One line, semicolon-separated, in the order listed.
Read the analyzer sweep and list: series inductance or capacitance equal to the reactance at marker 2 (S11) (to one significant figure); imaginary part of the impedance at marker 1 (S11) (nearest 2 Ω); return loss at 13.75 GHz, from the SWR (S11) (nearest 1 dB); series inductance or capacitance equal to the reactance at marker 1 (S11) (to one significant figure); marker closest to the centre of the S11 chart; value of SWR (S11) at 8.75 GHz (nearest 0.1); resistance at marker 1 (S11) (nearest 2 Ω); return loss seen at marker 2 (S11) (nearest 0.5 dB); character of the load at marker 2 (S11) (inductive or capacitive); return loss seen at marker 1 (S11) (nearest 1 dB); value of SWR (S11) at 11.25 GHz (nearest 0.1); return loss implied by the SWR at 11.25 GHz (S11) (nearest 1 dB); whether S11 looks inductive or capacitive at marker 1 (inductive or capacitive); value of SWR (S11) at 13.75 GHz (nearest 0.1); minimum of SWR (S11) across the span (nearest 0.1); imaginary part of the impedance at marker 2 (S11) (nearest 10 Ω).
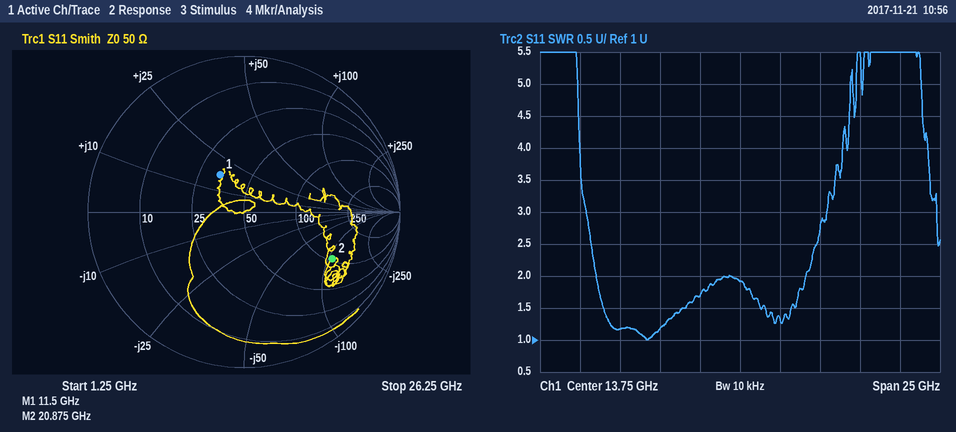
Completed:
70 fF; +18 Ω; 10 dB; 200 pH; marker 1; 1.2; 34 Ω; 4.0 dB; capacitive; 11 dB; 1.7; 12 dB; inductive; 1.9; 1.0; -110 Ω
